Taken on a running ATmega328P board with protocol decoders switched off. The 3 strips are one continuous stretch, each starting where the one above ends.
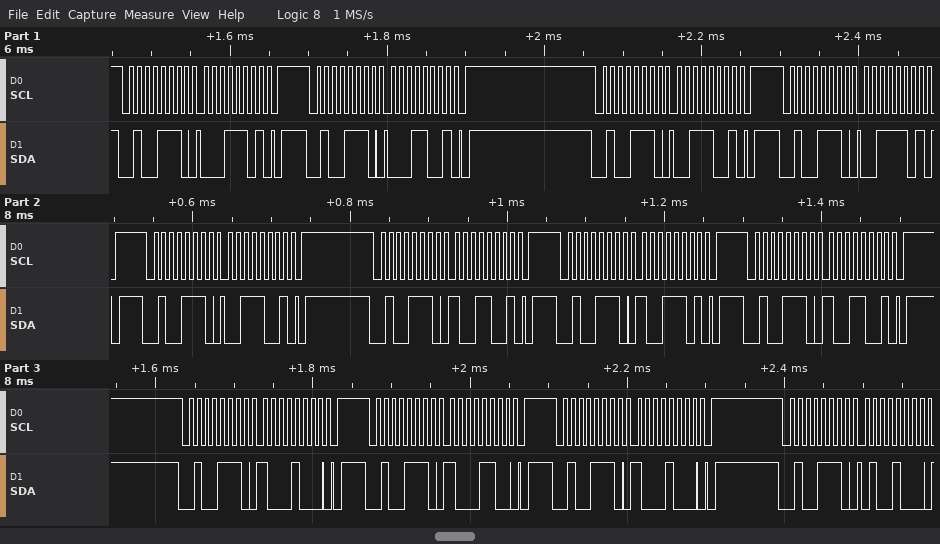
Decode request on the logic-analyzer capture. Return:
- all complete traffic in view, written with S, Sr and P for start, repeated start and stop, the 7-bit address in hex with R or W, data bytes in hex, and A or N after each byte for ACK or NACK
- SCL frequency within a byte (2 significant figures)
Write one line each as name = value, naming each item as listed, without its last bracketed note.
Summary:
all complete traffic in view, written with S, Sr and P for start, repeated start and stop, the 7-bit address in hex with R or W, data bytes in hex, and A or N after each byte for ACK or NACK = S 27W A 1D A P S 27W A 19 A P S 27W A 39 A P S 27W A 3D A P S 27W A 39 A P S 27W A 99 A P S 27W A 9D A P S 27W A 99 A P S 27W A 88 A P S 27W A 8C A P S 27W A 88 A P S 27W A 48 A
SCL frequency within a byte = 100 kHz
